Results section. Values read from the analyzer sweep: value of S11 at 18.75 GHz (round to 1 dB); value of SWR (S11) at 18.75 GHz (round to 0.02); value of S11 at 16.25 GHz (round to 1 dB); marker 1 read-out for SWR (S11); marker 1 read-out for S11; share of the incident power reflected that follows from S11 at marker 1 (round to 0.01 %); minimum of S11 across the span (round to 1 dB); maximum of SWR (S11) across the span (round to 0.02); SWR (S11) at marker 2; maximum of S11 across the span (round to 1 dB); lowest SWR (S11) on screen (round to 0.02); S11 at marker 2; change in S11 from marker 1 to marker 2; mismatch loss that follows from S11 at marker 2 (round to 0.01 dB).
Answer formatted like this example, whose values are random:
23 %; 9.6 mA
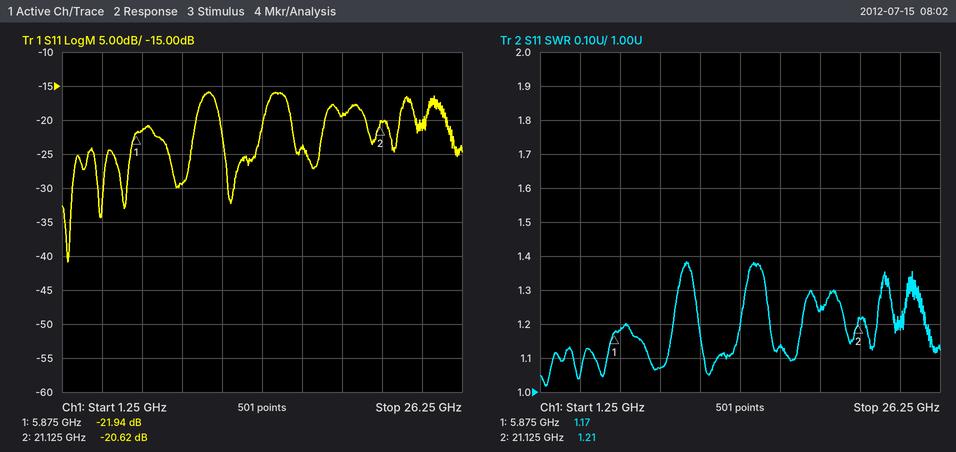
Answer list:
-19 dB; 1.24; -24 dB; 1.17; -21.94 dB; 0.64 %; -41 dB; 1.38; 1.21; -16 dB; 1.02; -20.62 dB; 1.32 dB; 0.04 dB
